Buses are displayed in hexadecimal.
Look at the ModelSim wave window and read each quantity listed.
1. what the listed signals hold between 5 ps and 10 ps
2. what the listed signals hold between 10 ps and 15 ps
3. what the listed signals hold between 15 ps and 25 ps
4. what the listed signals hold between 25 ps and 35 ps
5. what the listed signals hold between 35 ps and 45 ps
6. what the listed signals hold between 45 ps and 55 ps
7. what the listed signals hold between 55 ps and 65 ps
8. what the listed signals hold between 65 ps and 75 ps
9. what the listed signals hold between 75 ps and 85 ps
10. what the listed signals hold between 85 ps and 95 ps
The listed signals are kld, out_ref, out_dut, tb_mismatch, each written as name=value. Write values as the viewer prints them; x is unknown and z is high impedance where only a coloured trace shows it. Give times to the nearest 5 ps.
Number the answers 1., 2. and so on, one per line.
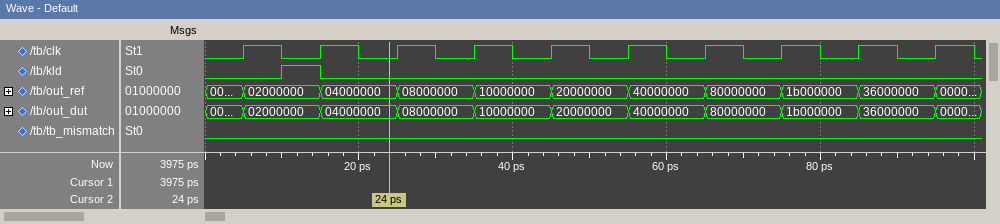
1. kld=0, out_ref=02000000, out_dut=02000000, tb_mismatch=0
2. kld=1, out_ref=02000000, out_dut=02000000, tb_mismatch=0
3. kld=0, out_ref=04000000, out_dut=04000000, tb_mismatch=0
4. kld=0, out_ref=08000000, out_dut=08000000, tb_mismatch=0
5. kld=0, out_ref=10000000, out_dut=10000000, tb_mismatch=0
6. kld=0, out_ref=20000000, out_dut=20000000, tb_mismatch=0
7. kld=0, out_ref=40000000, out_dut=40000000, tb_mismatch=0
8. kld=0, out_ref=80000000, out_dut=80000000, tb_mismatch=0
9. kld=0, out_ref=1b000000, out_dut=1b000000, tb_mismatch=0
10. kld=0, out_ref=36000000, out_dut=36000000, tb_mismatch=0
